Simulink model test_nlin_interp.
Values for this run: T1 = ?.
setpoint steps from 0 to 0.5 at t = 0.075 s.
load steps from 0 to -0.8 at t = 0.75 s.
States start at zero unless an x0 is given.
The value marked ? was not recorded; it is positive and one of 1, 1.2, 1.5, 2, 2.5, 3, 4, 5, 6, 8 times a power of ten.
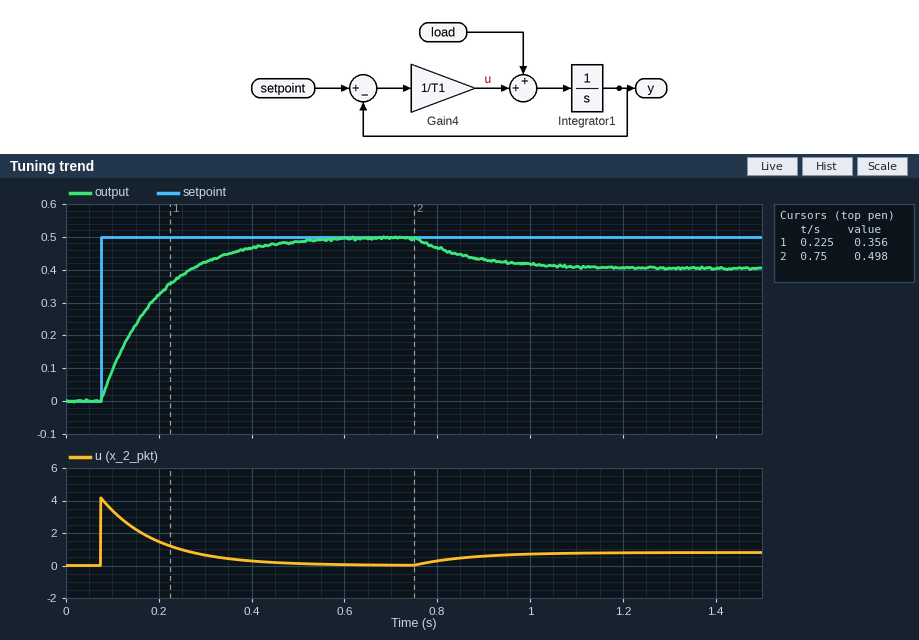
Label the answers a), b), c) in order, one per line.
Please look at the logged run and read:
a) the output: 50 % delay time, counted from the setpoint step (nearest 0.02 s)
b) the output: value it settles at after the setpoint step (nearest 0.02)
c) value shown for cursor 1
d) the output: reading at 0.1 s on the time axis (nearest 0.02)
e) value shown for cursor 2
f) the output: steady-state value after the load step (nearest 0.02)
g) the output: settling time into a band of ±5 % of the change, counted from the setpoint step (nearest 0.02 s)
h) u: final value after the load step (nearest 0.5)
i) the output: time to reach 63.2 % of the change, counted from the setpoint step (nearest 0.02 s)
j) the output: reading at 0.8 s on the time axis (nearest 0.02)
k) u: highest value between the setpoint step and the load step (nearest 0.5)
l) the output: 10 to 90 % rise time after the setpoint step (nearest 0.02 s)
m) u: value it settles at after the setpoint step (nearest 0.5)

a) 0.08 s
b) 0.50
c) 0.356
d) 0.10
e) 0.498
f) 0.40
g) 0.36 s
h) 1.0
i) 0.12 s
j) 0.46
k) 4.0
l) 0.26 s
m) 0.0
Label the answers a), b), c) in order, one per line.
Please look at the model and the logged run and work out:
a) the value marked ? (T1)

a) 0.12
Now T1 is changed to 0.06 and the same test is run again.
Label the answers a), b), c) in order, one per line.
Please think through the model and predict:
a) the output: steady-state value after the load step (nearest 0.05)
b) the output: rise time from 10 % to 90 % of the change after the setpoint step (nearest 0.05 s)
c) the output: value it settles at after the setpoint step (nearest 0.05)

a) 0.45
b) 0.15 s
c) 0.50
